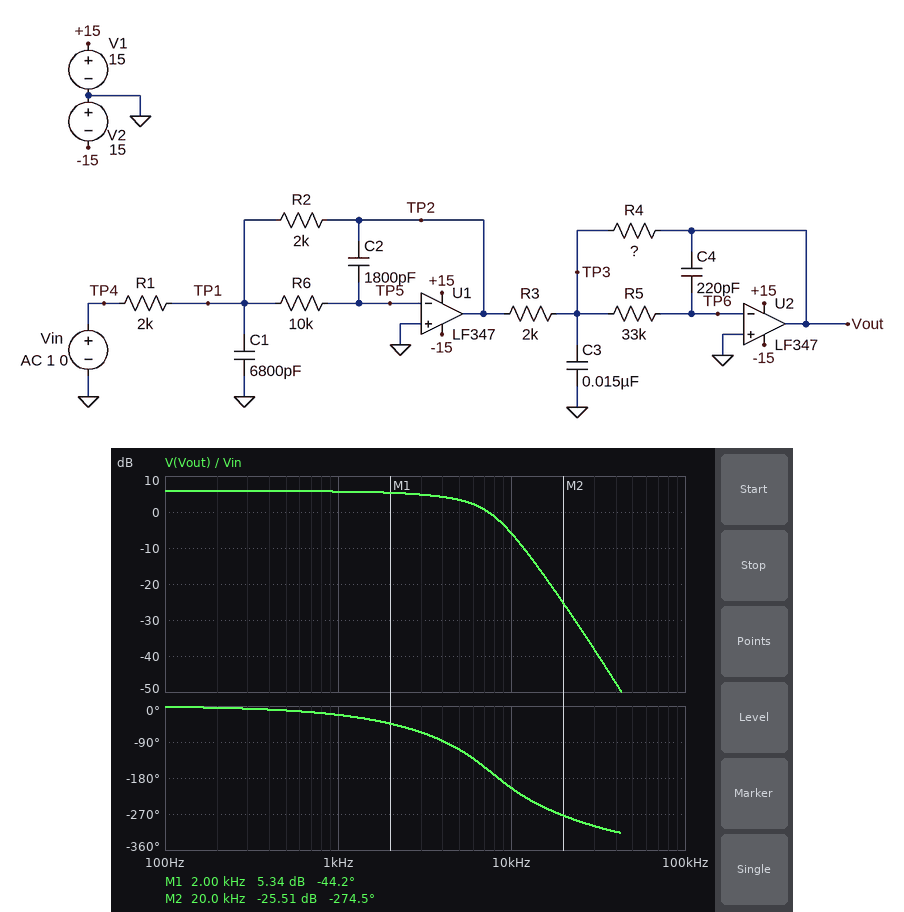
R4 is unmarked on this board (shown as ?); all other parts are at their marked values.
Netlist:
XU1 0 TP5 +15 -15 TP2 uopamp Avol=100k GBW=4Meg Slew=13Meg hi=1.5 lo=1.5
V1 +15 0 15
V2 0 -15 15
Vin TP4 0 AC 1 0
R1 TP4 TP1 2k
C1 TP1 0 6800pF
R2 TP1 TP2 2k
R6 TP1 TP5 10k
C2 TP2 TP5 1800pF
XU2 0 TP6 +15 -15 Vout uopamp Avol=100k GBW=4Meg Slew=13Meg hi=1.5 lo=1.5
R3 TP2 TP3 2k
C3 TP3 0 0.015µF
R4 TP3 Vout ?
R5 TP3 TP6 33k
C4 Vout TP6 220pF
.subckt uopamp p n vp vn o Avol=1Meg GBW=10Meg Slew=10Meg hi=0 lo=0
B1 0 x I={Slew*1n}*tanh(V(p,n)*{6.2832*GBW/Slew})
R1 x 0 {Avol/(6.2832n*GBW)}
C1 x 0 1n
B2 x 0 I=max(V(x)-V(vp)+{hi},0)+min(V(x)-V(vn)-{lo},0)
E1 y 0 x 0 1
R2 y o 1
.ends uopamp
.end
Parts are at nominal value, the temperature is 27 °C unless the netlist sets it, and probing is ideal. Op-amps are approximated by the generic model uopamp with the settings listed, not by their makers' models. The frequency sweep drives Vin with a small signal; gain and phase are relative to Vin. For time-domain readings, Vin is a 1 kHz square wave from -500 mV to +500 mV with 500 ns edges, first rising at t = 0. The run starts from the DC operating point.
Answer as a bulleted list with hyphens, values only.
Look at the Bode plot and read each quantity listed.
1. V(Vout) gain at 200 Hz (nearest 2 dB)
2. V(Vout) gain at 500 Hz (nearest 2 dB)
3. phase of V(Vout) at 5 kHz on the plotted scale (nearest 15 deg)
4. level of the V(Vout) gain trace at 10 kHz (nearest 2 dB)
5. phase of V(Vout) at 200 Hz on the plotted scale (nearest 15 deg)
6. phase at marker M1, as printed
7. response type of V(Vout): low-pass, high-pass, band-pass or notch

- 6 dB
- 6 dB
- -105 deg
- -6 dB
- 0 deg
- -44.2 deg
- low-pass
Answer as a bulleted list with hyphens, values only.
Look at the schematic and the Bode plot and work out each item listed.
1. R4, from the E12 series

- 3.9 kΩ
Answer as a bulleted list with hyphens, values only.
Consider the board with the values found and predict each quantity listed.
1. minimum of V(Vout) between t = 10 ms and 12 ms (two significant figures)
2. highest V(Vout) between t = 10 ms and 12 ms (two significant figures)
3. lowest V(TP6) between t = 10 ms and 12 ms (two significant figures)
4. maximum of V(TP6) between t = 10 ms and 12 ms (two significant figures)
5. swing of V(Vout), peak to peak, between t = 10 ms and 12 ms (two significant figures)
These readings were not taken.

- -980 mV
- 980 mV
- -1.2 mV
- 1.2 mV
- 2.0 V
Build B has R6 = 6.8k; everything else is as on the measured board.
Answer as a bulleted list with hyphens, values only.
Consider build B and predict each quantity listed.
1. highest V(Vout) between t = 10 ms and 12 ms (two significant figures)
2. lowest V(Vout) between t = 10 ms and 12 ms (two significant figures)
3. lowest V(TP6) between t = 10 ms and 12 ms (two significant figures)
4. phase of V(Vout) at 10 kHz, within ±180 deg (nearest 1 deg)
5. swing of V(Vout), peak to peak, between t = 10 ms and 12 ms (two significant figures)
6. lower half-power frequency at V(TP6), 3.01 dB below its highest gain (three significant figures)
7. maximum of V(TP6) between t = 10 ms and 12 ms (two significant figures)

- 1.1 V
- -1.1 V
- -1.4 mV
- 165 deg
- 2.2 V
- 3.68 kHz
- 1.4 mV
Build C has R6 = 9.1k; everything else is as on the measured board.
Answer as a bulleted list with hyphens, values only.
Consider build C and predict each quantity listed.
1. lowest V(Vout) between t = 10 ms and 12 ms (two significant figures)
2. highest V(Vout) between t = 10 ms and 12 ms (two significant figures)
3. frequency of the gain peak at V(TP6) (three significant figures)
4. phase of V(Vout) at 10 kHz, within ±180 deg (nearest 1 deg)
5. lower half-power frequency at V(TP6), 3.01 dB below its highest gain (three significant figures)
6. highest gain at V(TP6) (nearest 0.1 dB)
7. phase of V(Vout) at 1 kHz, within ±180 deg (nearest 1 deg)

- -1.0 V
- 1.0 V
- 6.24 kHz
- 157 deg
- 3.30 kHz
- -53.7 dB
- -21 deg
